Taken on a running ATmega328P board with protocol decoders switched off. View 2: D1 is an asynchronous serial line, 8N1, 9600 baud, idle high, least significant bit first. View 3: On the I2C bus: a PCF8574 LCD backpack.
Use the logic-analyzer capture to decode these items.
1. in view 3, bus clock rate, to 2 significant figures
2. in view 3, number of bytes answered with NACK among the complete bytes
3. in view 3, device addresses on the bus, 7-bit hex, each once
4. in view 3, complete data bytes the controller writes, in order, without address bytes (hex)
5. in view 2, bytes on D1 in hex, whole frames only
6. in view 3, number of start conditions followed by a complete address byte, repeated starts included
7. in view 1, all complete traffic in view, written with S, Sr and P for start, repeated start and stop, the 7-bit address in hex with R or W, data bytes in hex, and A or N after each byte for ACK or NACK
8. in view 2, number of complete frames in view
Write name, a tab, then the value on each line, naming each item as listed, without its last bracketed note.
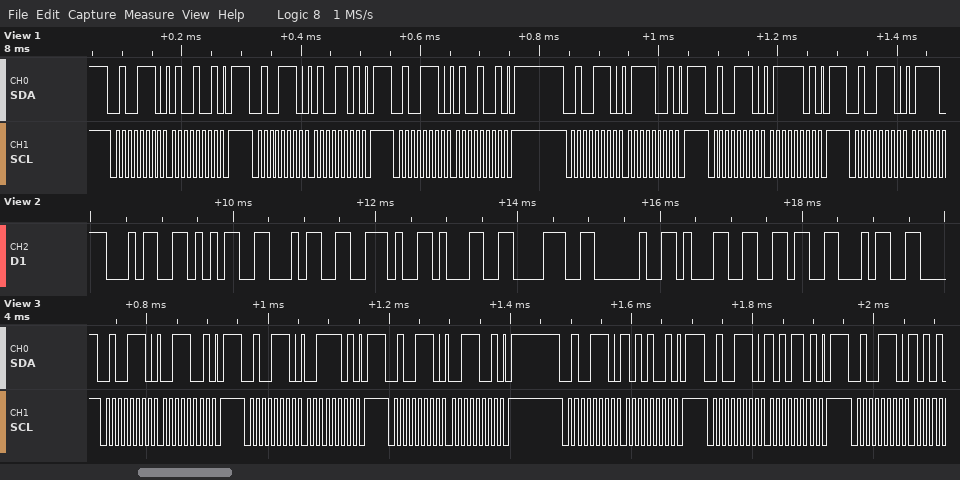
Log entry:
in view 3, bus clock rate, to 2 significant figures	100 kHz
in view 3, number of bytes answered with NACK among the complete bytes	0
in view 3, device addresses on the bus, 7-bit hex, each once	0x27
in view 3, complete data bytes the controller writes, in order, without address bytes	39 3D 39 A9 AD
in view 2, bytes on D1 in hex, whole frames only	34 35 34 2E 31 38 20 31 36 34
in view 3, number of start conditions followed by a complete address byte, repeated starts included	6
in view 1, all complete traffic in view, written with S, Sr and P for start, repeated start and stop, the 7-bit address in hex with R or W, data bytes in hex, and A or N after each byte for ACK or NACK	S 27W A 49 A P S 27W A 4D A P S 27W A 49 A P S 27W A 79 A P S 27W A 7D A P S 27W A
in view 2, number of complete frames in view	10
